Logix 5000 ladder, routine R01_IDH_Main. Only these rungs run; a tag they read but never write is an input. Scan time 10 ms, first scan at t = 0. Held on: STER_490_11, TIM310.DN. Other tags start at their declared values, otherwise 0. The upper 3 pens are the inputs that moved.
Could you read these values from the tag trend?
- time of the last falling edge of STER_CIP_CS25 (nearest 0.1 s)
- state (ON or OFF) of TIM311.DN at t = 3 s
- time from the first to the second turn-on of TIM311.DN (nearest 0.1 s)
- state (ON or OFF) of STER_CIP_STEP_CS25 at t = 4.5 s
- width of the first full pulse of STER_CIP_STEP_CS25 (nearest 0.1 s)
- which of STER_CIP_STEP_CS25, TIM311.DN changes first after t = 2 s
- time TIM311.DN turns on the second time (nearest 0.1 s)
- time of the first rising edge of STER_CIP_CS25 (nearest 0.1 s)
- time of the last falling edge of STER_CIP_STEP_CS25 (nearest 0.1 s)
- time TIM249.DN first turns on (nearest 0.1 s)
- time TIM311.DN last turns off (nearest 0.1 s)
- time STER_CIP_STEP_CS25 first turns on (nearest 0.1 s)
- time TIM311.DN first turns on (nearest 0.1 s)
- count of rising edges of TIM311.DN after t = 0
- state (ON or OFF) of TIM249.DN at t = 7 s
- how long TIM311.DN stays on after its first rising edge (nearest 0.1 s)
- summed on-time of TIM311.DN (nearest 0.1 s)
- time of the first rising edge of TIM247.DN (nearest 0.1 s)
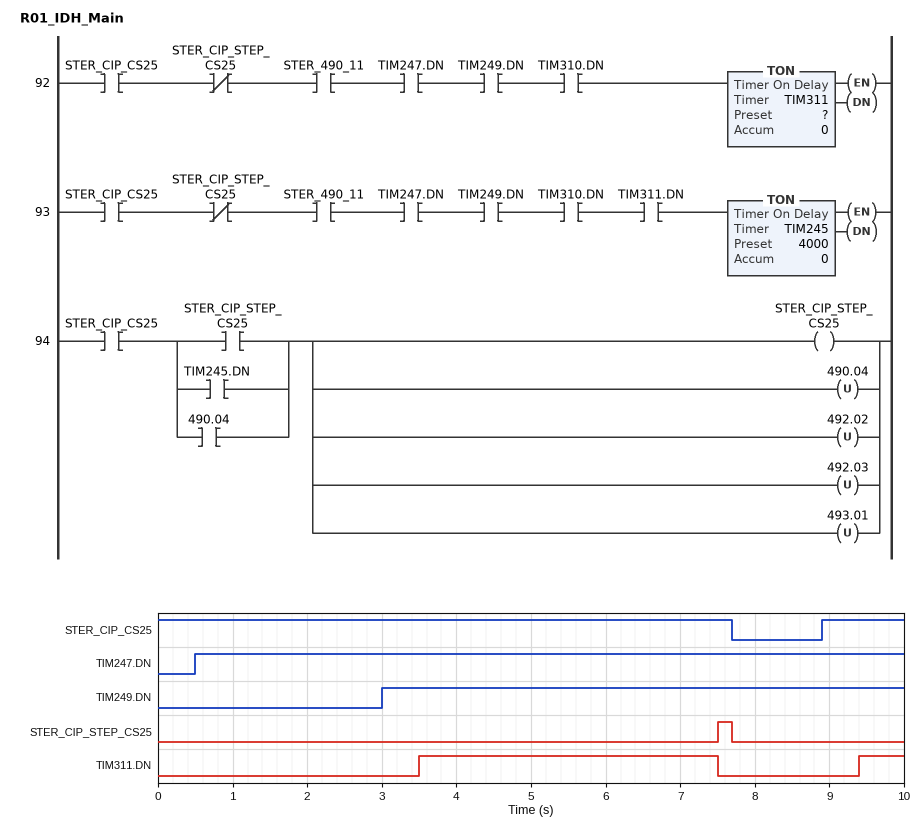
7.7 s
OFF
5.9 s
OFF
0.2 s
TIM311.DN
9.4 s
8.9 s
7.7 s
3.0 s
7.5 s
7.5 s
3.5 s
2
ON
4.0 s
4.6 s
0.5 s
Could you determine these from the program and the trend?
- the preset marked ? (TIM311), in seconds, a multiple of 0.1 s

0.5 s
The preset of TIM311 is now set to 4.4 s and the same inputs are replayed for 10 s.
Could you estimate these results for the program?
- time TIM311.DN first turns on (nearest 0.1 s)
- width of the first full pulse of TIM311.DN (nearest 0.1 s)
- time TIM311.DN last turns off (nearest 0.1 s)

7.4 s
0.3 s
7.7 s
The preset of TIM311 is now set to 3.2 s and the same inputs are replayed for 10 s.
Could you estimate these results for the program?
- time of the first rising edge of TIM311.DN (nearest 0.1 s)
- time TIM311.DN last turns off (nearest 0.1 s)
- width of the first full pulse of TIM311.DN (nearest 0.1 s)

6.2 s
7.7 s
1.5 s
